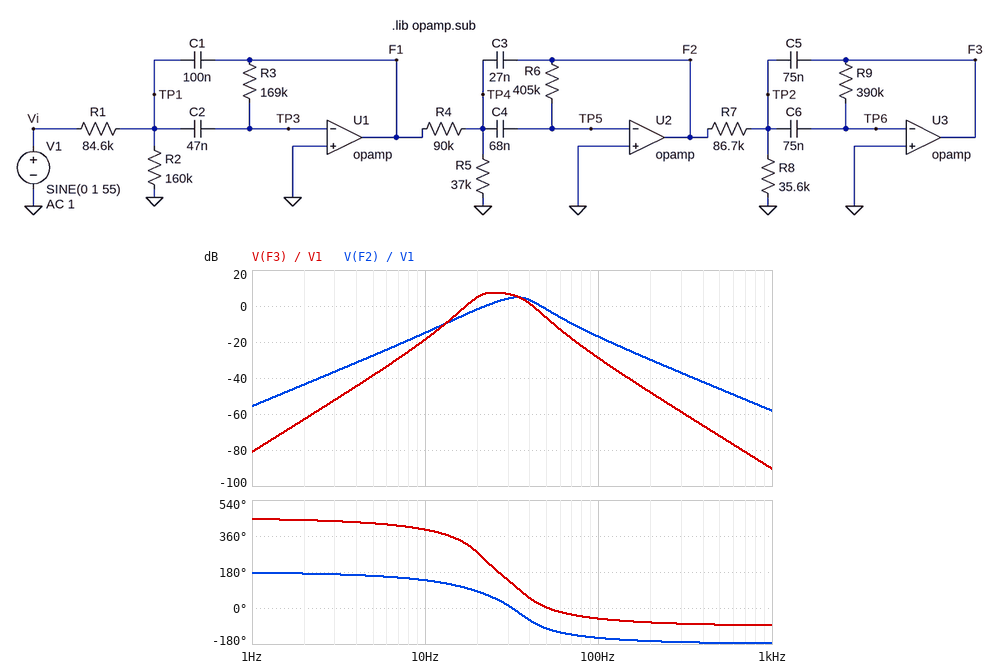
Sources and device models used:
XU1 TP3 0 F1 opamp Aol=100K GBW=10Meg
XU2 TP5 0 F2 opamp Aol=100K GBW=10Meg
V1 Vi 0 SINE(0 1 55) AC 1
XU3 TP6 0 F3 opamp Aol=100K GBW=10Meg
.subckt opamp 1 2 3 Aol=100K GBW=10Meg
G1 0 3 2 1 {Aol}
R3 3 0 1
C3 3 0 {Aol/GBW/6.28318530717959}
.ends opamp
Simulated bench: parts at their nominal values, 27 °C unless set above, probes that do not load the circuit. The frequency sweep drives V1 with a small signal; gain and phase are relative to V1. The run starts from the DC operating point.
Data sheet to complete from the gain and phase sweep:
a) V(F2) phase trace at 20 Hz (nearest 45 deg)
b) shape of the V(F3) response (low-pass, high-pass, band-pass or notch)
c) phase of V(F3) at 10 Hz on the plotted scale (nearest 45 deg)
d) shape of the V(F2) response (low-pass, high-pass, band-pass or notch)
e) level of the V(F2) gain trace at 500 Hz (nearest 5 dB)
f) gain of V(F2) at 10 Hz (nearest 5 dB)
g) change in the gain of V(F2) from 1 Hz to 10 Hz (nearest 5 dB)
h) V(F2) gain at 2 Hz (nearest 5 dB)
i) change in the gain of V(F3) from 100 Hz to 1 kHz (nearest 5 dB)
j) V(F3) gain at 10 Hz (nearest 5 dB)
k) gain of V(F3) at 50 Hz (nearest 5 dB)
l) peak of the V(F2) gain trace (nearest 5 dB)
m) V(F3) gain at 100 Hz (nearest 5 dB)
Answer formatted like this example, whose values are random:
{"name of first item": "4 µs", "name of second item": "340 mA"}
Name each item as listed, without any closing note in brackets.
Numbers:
{"V(F2) phase trace at 20 Hz": "90 deg", "shape of the V(F3) response": "band-pass", "phase of V(F3) at 10 Hz on the plotted scale": "405 deg", "shape of the V(F2) response": "band-pass", "level of the V(F2) gain trace at 500 Hz": "-45 dB", "gain of V(F2) at 10 Hz": "-15 dB", "change in the gain of V(F2) from 1 Hz to 10 Hz": "40 dB", "V(F2) gain at 2 Hz": "-45 dB", "change in the gain of V(F3) from 100 Hz to 1 kHz": "-60 dB", "V(F3) gain at 10 Hz": "-20 dB", "gain of V(F3) at 50 Hz": "-5 dB", "peak of the V(F2) gain trace": "5 dB", "V(F3) gain at 100 Hz": "-30 dB"}
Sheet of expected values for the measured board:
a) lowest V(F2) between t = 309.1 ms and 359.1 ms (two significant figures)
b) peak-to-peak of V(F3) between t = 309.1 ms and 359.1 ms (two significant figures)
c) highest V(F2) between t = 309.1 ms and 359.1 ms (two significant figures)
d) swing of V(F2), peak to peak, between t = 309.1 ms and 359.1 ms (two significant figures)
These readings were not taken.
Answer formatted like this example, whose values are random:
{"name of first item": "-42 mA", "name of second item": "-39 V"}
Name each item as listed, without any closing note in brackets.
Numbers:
{"lowest V(F2) between t = 309.1 ms and 359.1 ms": "-620 mV", "peak-to-peak of V(F3) between t = 309.1 ms and 359.1 ms": "630 mV", "highest V(F2) between t = 309.1 ms and 359.1 ms": "620 mV", "swing of V(F2), peak to peak, between t = 309.1 ms and 359.1 ms": "1.2 V"}
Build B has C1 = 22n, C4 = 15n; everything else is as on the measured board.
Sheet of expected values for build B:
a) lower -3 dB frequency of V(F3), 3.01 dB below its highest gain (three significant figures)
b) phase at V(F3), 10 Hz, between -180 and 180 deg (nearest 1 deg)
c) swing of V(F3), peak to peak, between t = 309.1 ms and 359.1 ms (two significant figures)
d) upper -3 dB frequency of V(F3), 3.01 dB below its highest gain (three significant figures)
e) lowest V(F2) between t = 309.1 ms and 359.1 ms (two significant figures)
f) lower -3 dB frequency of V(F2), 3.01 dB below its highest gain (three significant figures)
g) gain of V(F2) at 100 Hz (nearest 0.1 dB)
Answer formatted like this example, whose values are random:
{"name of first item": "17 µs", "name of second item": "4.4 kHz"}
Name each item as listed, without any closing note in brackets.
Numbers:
{"lower -3 dB frequency of V(F3), 3.01 dB below its highest gain": "27.8 Hz", "phase at V(F3), 10 Hz, between -180 and 180 deg": "55 deg", "swing of V(F3), peak to peak, between t = 309.1 ms and 359.1 ms": "1.4 V", "upper -3 dB frequency of V(F3), 3.01 dB below its highest gain": "83.1 Hz", "lowest V(F2) between t = 309.1 ms and 359.1 ms": "-1.3 V", "lower -3 dB frequency of V(F2), 3.01 dB below its highest gain": "54.3 Hz", "gain of V(F2) at 100 Hz": "0 dB"}
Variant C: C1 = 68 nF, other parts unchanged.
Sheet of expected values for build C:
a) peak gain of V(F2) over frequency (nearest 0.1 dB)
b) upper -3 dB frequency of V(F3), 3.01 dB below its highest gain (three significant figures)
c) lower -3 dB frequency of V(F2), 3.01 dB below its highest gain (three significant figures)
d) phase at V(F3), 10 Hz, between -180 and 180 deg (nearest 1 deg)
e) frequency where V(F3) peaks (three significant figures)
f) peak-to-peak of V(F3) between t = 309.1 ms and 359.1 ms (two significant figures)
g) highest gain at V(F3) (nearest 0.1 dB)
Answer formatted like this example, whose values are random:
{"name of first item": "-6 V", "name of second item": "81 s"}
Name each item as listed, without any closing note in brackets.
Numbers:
{"peak gain of V(F2) over frequency": "7.9 dB", "upper -3 dB frequency of V(F3), 3.01 dB below its highest gain": "37.5 Hz", "lower -3 dB frequency of V(F2), 3.01 dB below its highest gain": "26.7 Hz", "phase at V(F3), 10 Hz, between -180 and 180 deg": "39 deg", "frequency where V(F3) peaks": "27.3 Hz", "peak-to-peak of V(F3) between t = 309.1 ms and 359.1 ms": "950 mV", "highest gain at V(F3)": "9.5 dB"}
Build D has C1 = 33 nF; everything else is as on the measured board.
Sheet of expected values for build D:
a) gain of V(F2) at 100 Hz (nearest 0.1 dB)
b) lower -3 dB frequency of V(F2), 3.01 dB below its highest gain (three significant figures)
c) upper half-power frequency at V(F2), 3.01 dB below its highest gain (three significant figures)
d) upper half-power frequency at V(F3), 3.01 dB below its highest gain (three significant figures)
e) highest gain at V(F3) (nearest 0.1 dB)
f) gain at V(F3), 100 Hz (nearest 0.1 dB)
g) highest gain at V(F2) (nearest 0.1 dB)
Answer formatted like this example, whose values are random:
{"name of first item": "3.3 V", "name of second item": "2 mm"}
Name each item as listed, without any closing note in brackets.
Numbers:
{"gain of V(F2) at 100 Hz": "-7.2 dB", "lower -3 dB frequency of V(F2), 3.01 dB below its highest gain": "29.4 Hz", "upper half-power frequency at V(F2), 3.01 dB below its highest gain": "47.6 Hz", "upper half-power frequency at V(F3), 3.01 dB below its highest gain": "41.1 Hz", "highest gain at V(F3)": "11.4 dB", "gain at V(F3), 100 Hz": "-19.1 dB", "highest gain at V(F2)": "11.3 dB"}
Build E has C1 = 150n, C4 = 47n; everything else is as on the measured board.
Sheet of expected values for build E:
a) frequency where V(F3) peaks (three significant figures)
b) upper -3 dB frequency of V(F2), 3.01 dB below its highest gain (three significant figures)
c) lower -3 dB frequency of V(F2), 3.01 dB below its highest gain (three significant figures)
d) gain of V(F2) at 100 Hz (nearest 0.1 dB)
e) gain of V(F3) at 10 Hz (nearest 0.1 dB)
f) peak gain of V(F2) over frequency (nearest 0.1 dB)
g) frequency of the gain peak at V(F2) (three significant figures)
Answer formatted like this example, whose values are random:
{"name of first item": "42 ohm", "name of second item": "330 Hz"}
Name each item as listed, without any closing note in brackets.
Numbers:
{"frequency where V(F3) peaks": "23.3 Hz", "upper -3 dB frequency of V(F2), 3.01 dB below its highest gain": "50.9 Hz", "lower -3 dB frequency of V(F2), 3.01 dB below its highest gain": "27.9 Hz", "gain of V(F2) at 100 Hz": "-20.2 dB", "gain of V(F3) at 10 Hz": "-22.2 dB", "peak gain of V(F2) over frequency": "-1.4 dB", "frequency of the gain peak at V(F2)": "40.4 Hz"}
